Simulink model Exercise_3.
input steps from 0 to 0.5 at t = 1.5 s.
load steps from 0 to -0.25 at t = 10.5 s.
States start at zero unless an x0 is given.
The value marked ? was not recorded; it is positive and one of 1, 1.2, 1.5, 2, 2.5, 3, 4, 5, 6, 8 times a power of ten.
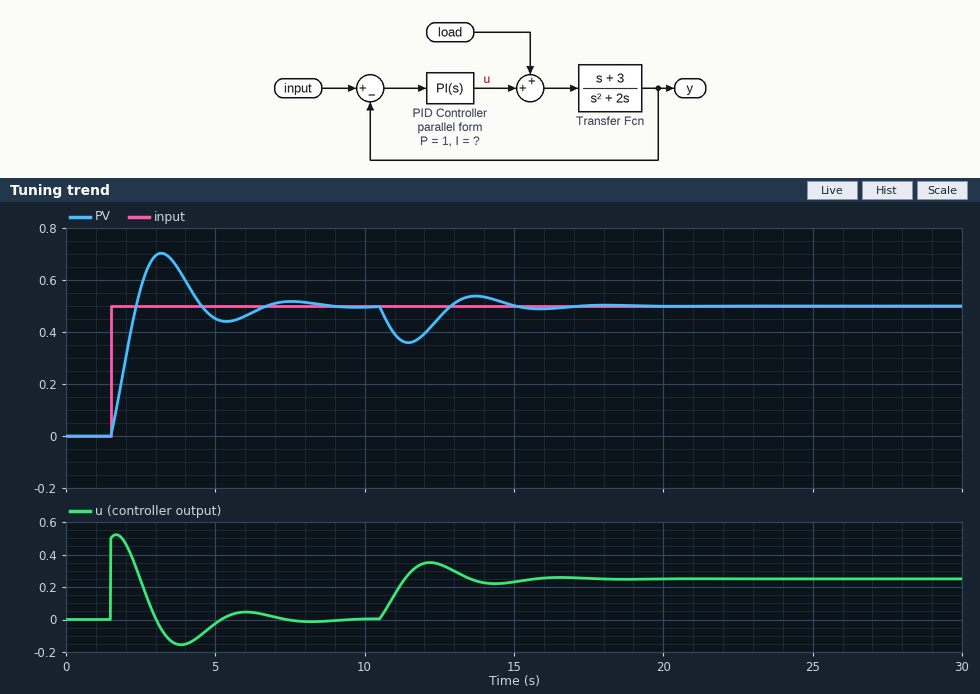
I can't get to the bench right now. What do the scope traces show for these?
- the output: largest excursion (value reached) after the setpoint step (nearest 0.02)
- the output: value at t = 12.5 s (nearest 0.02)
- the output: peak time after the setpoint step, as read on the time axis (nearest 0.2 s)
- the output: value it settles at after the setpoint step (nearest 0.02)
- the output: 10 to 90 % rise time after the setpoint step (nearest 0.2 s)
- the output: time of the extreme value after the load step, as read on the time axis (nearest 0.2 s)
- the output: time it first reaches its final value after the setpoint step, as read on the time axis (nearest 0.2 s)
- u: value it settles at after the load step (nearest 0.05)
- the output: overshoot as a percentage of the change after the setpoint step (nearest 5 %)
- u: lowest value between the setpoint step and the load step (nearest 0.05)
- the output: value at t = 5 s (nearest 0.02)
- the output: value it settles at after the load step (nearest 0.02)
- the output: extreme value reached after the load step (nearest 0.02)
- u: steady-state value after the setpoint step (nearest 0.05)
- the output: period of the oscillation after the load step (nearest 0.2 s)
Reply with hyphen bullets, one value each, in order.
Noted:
- 0.70
- 0.46
- 3.2 s
- 0.50
- 0.6 s
- 11.4 s
- 2.4 s
- 0.25
- 40 %
- -0.15
- 0.46
- 0.50
- 0.36
- 0.00
- 4.4 s
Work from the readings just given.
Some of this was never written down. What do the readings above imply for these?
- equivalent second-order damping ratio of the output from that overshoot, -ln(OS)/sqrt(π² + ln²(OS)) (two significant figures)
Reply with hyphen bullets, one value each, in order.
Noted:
- 0.28
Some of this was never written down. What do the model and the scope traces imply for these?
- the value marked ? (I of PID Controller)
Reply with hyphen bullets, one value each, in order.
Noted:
- 1.5
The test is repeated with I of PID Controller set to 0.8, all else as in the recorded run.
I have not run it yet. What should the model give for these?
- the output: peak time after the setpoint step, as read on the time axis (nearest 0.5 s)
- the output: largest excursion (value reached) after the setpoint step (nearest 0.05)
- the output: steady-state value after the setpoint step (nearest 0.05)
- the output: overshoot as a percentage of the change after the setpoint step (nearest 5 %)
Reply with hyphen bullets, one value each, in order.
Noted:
- 3.5 s
- 0.65
- 0.50
- 30 %
